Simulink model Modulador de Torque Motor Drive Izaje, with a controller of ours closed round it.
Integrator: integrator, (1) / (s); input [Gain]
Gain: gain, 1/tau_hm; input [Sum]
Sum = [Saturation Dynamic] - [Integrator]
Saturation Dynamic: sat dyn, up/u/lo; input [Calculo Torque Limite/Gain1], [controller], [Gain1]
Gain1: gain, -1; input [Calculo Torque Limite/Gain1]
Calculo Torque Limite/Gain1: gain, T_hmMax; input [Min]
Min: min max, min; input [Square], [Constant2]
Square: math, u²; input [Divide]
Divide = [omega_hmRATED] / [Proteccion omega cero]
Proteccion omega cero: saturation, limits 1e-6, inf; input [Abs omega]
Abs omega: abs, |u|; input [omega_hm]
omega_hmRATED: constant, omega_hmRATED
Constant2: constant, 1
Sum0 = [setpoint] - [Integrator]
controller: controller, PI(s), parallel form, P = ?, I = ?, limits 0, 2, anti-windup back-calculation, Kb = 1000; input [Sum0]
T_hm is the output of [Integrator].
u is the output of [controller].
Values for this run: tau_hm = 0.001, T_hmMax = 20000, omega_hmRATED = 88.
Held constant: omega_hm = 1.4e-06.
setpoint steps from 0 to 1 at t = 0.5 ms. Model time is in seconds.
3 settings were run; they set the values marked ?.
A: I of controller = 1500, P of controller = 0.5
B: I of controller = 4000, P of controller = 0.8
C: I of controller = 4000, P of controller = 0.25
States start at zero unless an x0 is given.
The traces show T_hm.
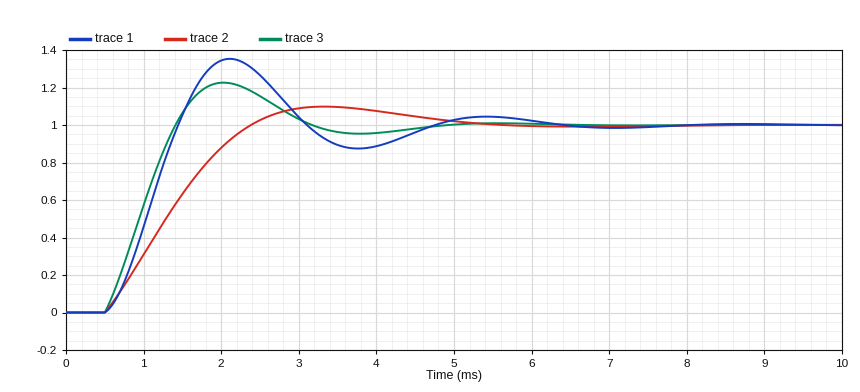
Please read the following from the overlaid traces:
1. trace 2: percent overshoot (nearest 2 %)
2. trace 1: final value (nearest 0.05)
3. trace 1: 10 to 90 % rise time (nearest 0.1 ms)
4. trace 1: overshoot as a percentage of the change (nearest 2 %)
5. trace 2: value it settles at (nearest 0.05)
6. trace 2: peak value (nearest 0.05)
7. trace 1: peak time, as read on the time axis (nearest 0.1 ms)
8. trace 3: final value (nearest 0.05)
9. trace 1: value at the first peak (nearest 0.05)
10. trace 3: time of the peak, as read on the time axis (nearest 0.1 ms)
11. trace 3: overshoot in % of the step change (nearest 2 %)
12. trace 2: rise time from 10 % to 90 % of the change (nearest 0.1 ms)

10 %
1.00
0.7 ms
36 %
1.00
1.10
2.1 ms
1.00
1.35
2.0 ms
22 %
1.4 ms
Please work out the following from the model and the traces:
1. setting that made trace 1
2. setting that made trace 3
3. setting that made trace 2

C
B
A
